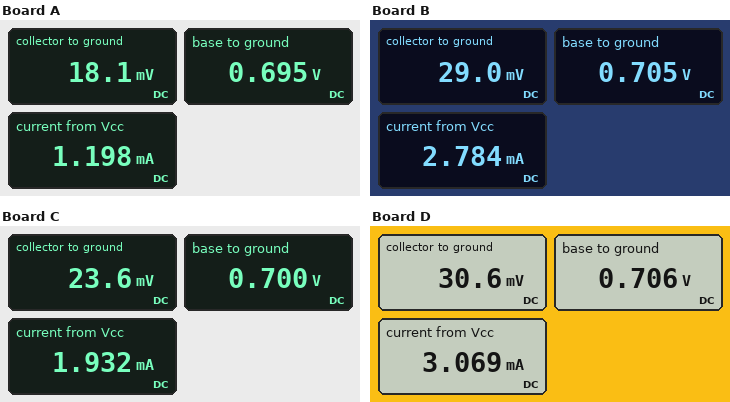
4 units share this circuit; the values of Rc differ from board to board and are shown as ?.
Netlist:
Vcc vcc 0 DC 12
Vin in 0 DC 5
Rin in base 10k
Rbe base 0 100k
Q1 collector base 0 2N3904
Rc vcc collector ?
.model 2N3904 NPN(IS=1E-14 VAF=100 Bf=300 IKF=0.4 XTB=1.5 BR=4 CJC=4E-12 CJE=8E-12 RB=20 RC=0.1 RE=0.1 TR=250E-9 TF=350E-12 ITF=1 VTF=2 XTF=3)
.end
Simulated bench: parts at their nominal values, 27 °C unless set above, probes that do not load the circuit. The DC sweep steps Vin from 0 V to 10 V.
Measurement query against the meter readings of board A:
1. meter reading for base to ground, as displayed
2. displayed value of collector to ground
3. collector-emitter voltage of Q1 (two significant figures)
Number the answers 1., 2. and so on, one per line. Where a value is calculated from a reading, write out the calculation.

1. 0.695 V
2. 18.1 mV
3. 18.1 mV = 18 mV
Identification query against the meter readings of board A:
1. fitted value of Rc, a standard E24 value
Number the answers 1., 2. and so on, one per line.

1. 10 kΩ
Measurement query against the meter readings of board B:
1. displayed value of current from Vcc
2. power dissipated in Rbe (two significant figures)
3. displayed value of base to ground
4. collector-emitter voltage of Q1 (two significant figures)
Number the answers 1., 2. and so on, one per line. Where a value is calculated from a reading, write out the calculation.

1. 2.784 mA
2. (705 mV)^2 / 100 kΩ = 5.0 µW
3. 0.705 V
4. 29 mV = 29 mV
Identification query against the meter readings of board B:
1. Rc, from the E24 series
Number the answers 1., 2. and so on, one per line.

1. 4.3 kΩ
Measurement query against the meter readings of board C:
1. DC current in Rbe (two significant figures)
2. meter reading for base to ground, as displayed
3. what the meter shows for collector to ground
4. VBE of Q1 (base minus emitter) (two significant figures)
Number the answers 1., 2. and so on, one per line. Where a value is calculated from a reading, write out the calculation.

1. (700 mV) / 100 kΩ = 7.0 µA
2. 0.700 V
3. 23.6 mV
4. 700 mV = 700 mV
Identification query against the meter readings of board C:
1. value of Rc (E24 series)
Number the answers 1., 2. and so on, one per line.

1. 6.2 kΩ
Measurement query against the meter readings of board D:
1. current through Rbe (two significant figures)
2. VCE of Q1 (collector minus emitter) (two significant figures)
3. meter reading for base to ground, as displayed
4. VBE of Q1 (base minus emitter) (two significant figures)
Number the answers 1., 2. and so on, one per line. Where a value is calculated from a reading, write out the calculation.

1. (706 mV) / 100 kΩ = 7.1 µA
2. 30.6 mV = 31 mV
3. 0.706 V
4. 706 mV = 710 mV
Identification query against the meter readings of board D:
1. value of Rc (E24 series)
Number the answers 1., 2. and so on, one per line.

1. 3.9 kΩ
